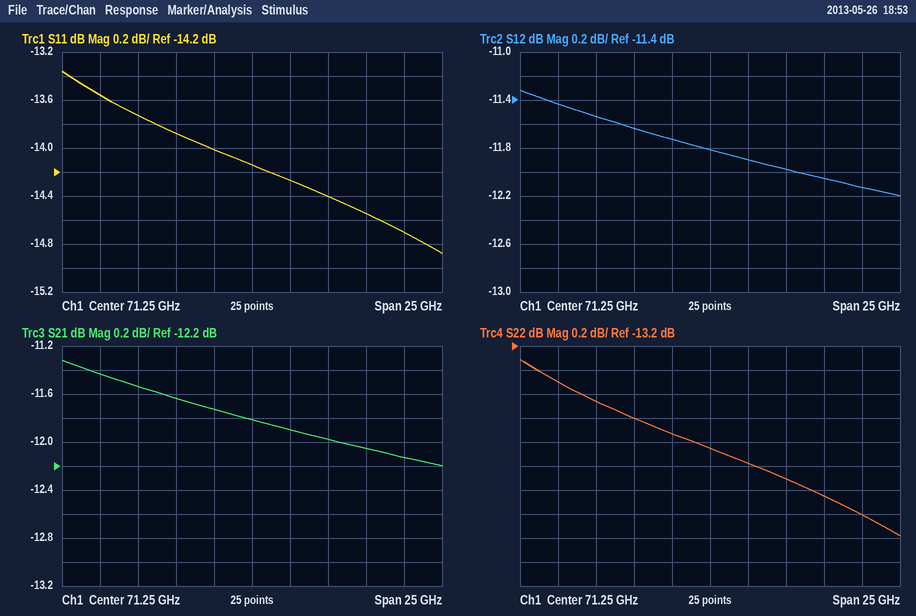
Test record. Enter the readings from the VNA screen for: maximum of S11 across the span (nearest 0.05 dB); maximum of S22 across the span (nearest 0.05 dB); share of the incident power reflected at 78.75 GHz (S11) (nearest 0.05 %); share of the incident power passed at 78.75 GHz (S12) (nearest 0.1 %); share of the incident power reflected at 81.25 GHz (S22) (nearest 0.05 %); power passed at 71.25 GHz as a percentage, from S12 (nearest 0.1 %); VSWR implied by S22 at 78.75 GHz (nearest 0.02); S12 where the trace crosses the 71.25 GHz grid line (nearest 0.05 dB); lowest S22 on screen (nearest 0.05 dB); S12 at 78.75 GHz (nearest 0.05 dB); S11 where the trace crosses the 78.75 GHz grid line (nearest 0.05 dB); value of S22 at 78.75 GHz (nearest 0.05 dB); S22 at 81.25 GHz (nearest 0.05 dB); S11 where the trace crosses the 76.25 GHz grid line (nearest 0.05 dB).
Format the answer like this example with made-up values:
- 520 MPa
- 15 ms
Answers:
- -13.35 dB
- -13.30 dB
- 3.50 %
- 6.2 %
- 3.45 %
- 6.6 %
- 1.46
- -11.80 dB
- -14.80 dB
- -12.05 dB
- -14.55 dB
- -14.45 dB
- -14.60 dB
- -14.40 dB
